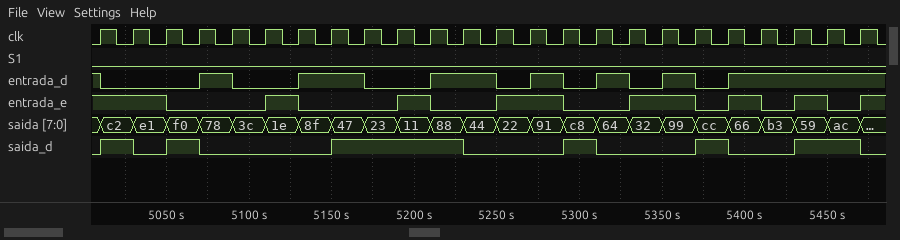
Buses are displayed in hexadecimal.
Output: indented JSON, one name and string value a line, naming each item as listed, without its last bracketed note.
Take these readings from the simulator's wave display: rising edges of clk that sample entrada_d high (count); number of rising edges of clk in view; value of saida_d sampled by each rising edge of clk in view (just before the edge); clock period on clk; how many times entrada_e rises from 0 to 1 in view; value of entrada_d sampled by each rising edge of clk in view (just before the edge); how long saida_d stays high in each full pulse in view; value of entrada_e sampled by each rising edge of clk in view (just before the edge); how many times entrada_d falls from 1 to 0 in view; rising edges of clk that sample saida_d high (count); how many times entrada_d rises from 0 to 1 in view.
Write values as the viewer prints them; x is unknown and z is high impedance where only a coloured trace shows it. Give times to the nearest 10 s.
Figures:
{
  "rising edges of clk that sample entrada_d high": "13",
  "number of rising edges of clk in view": "24",
  "value of saida_d sampled by each rising edge of clk in view": "0 1 0 1 0 0 0 0 1 1 1 1 0 0 0 1 0 0 0 1 0 0 1 1",
  "clock period on clk": "20 s",
  "how many times entrada_e rises from 0 to 1 in view": "7",
  "value of entrada_d sampled by each rising edge of clk in view": "1 0 0 0 1 0 0 1 1 0 0 1 1 0 1 0 1 0 1 0 1 1 1 1",
  "how long saida_d stays high in each full pulse in view": "20 s, 20 s, 80 s, 20 s, 20 s, 40 s",
  "value of entrada_e sampled by each rising edge of clk in view": "1 1 1 0 0 0 1 0 0 0 1 0 0 1 1 0 0 1 1 0 1 0 1 0",
  "how many times entrada_d falls from 1 to 0 in view": "7",
  "rising edges of clk that sample saida_d high": "10",
  "how many times entrada_d rises from 0 to 1 in view": "7"
}
